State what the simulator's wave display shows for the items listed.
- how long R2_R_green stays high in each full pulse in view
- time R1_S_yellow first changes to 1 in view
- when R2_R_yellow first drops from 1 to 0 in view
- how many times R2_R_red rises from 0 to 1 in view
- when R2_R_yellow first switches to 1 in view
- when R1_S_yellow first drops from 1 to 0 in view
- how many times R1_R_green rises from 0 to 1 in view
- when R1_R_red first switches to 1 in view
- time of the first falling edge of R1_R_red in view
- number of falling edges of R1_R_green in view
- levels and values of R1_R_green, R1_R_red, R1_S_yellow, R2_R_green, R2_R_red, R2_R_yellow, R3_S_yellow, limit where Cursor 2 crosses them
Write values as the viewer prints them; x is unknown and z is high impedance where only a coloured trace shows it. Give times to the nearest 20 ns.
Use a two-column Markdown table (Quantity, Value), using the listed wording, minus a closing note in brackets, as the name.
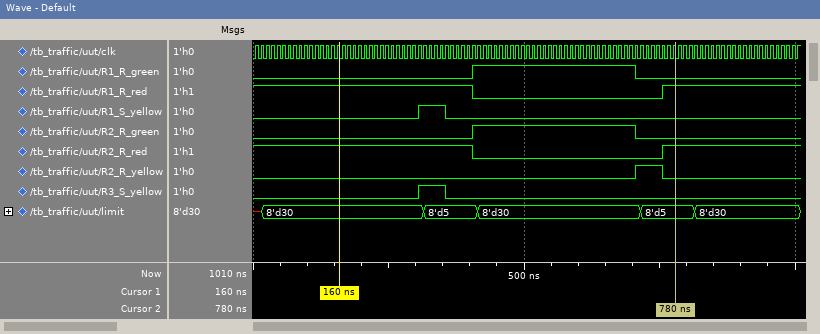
| Quantity | Value |
|---|---|
| how long R2_R_green stays high in each full pulse in view | 300 ns |
| time R1_S_yellow first changes to 1 in view | 300 ns |
| when R2_R_yellow first drops from 1 to 0 in view | 760 ns |
| how many times R2_R_red rises from 0 to 1 in view | 1 |
| when R2_R_yellow first switches to 1 in view | 700 ns |
| when R1_S_yellow first drops from 1 to 0 in view | 360 ns |
| how many times R1_R_green rises from 0 to 1 in view | 1 |
| when R1_R_red first switches to 1 in view | 760 ns |
| time of the first falling edge of R1_R_red in view | 400 ns |
| number of falling edges of R1_R_green in view | 1 |
| levels and values of R1_R_green, R1_R_red, R1_S_yellow, R2_R_green, R2_R_red, R2_R_yellow, R3_S_yellow, limit where Cursor 2 crosses them | R1_R_green=0, R1_R_red=1, R1_S_yellow=0, R2_R_green=0, R2_R_red=1, R2_R_yellow=0, R3_S_yellow=0, limit=8'd5 |
